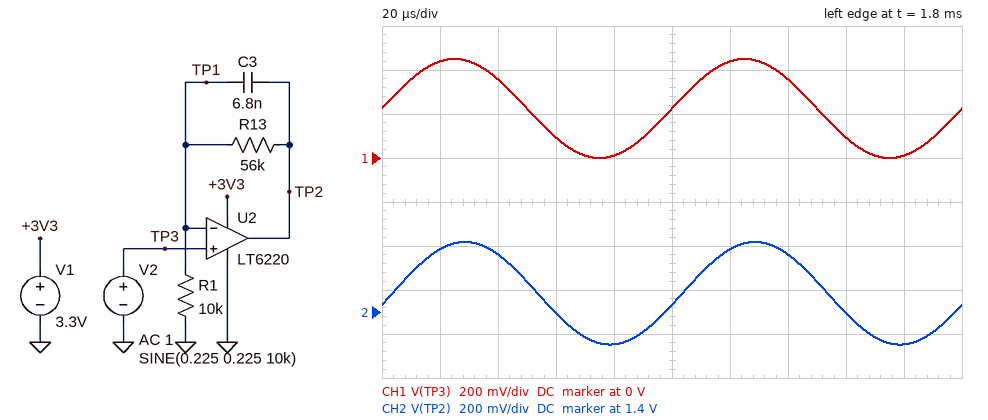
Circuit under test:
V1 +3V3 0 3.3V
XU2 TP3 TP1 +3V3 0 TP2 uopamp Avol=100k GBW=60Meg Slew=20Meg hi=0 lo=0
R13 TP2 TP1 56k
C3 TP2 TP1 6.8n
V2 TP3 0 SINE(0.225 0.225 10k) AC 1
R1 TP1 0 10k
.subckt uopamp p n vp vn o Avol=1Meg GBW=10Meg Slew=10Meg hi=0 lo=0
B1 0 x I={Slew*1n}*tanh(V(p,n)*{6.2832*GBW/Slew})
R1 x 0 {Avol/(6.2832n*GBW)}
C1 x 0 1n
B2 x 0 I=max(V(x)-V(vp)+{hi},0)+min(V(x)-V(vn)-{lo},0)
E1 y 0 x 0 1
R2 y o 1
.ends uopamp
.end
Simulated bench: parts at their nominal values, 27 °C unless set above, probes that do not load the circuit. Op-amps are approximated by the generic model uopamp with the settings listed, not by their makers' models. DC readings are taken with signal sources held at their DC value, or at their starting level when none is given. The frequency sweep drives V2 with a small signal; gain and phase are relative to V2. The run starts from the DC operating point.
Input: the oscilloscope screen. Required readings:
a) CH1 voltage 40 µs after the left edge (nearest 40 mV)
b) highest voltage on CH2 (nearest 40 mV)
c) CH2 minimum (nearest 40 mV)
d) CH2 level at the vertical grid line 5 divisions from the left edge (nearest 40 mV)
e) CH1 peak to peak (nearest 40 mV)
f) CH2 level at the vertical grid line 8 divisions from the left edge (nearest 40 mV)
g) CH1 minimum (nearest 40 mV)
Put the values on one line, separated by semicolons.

360 mV; 1.72 V; 1.24 V; 1.44 V; 440 mV; 1.40 V; 0 V
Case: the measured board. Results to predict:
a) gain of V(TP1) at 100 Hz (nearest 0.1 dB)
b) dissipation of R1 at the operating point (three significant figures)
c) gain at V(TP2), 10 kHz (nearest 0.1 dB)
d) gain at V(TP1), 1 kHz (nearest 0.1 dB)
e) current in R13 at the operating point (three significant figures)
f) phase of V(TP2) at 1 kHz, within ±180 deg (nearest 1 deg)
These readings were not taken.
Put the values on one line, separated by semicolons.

0 dB; 5.06 µW; 0.3 dB; 0 dB; 22.5 µA; -47 deg
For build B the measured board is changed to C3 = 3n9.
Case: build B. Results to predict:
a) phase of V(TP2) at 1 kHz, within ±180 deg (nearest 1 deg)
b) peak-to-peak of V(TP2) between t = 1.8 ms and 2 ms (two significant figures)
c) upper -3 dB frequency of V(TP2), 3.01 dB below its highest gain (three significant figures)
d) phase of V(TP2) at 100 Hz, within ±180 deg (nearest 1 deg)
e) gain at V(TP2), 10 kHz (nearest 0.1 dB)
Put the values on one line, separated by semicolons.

-42 deg; 500 mV; 746 Hz; -7 deg; 0.9 dB
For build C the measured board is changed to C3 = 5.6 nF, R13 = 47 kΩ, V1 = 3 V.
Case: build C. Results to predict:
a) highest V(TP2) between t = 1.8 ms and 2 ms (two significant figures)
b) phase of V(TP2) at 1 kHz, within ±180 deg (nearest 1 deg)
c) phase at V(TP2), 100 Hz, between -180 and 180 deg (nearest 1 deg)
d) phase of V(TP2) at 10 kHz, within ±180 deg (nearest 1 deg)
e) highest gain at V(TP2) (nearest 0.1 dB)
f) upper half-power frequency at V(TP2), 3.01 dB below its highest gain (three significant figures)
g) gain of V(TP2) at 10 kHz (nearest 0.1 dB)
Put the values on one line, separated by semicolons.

1.5 V; -43 deg; -8 deg; -16 deg; 15.1 dB; 624 Hz; 0.5 dB
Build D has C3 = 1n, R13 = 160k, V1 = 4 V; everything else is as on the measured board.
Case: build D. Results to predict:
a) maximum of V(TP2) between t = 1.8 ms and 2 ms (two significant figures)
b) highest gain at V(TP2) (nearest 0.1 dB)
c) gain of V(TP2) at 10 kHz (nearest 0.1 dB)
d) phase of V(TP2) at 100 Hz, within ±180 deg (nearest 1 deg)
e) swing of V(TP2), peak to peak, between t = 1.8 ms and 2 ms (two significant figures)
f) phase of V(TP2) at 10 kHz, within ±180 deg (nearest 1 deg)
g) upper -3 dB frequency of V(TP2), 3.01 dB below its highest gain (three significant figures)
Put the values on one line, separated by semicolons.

4.0 V; 24.6 dB; 5.8 dB; -5 deg; 790 mV; -54 deg; 998 Hz
